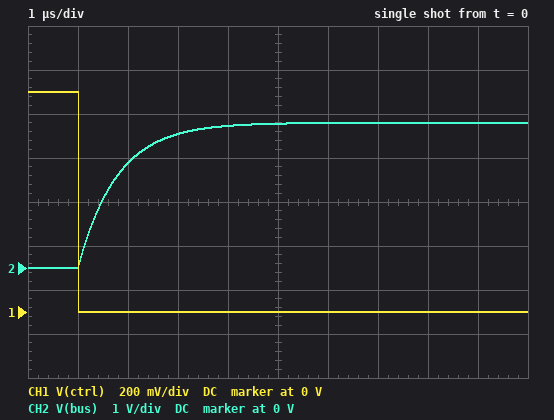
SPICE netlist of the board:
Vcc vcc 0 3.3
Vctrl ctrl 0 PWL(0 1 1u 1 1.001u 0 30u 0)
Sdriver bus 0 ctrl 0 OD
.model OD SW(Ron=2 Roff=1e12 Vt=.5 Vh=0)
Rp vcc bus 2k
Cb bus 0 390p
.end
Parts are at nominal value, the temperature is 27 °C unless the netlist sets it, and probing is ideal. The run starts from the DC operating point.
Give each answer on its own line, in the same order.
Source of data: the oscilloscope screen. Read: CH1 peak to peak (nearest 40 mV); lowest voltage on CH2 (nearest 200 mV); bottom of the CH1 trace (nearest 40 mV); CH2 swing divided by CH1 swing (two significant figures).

1.00 V
0 V
0 V
3.3
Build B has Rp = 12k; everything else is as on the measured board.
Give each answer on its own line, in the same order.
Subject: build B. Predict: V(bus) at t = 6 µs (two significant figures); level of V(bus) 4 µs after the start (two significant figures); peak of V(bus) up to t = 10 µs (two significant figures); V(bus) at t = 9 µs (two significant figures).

2.2 V
1.6 V
2.8 V
2.7 V
